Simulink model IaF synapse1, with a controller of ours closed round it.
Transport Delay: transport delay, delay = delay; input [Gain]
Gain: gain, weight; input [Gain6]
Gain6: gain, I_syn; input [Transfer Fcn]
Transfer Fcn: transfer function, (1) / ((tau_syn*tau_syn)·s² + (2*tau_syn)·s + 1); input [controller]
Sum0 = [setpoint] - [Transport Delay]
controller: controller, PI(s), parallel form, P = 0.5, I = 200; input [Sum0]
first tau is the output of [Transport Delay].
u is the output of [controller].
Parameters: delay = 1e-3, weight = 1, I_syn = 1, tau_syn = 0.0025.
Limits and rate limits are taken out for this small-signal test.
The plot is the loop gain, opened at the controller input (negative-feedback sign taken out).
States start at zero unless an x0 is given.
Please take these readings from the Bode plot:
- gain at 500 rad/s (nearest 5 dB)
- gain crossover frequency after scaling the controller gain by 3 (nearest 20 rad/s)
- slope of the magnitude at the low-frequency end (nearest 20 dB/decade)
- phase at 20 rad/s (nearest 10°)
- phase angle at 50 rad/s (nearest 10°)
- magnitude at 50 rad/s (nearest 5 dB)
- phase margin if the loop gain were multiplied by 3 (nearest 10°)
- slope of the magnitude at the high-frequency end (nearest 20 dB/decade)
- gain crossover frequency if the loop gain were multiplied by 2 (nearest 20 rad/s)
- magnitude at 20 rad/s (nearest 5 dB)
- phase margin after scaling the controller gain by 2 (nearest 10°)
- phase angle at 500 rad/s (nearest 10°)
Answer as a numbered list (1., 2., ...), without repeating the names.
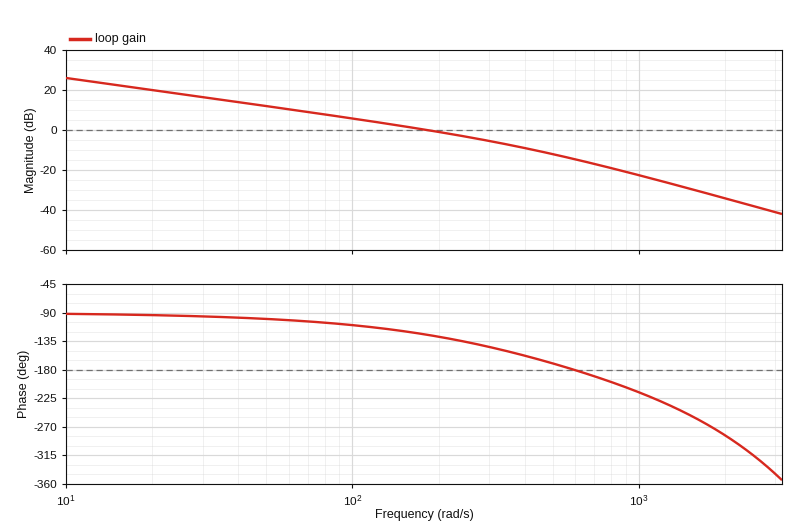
1. -10 dB
2. 420 rad/s
3. -20 dB/decade
4. -90°
5. -100°
6. 10 dB
7. 20°
8. -40 dB/decade
9. 320 rad/s
10. 20 dB
11. 30°
12. -170°
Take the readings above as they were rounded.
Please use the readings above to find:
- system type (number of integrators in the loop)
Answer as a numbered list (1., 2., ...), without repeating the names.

1. 1
